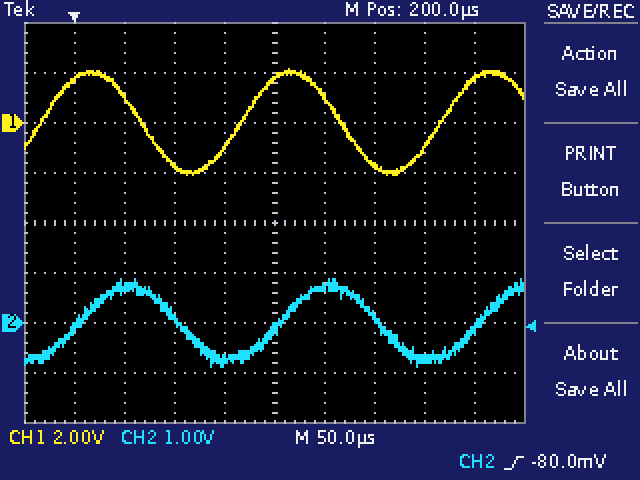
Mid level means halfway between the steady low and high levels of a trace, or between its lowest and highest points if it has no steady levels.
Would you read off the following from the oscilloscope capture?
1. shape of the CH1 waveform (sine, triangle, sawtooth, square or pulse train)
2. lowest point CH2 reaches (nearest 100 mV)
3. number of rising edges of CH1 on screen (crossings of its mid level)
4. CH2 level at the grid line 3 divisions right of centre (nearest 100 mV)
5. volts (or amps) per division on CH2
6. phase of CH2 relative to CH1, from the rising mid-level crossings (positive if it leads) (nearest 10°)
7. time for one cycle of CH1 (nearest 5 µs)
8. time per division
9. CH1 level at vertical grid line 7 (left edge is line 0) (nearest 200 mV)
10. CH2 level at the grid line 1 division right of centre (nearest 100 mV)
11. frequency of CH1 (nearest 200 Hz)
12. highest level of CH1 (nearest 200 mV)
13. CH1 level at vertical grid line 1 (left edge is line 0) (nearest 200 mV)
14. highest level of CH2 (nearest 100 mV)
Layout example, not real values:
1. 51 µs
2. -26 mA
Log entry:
1. sine
2. -900 mV
3. 3
4. -700 mV
5. 1 V
6. -70°
7. 200 µs
8. 50 µs
9. -1.6 V
10. 700 mV
11. 5.0 kHz
12. 2.2 V
13. 1.8 V
14. 900 mV
